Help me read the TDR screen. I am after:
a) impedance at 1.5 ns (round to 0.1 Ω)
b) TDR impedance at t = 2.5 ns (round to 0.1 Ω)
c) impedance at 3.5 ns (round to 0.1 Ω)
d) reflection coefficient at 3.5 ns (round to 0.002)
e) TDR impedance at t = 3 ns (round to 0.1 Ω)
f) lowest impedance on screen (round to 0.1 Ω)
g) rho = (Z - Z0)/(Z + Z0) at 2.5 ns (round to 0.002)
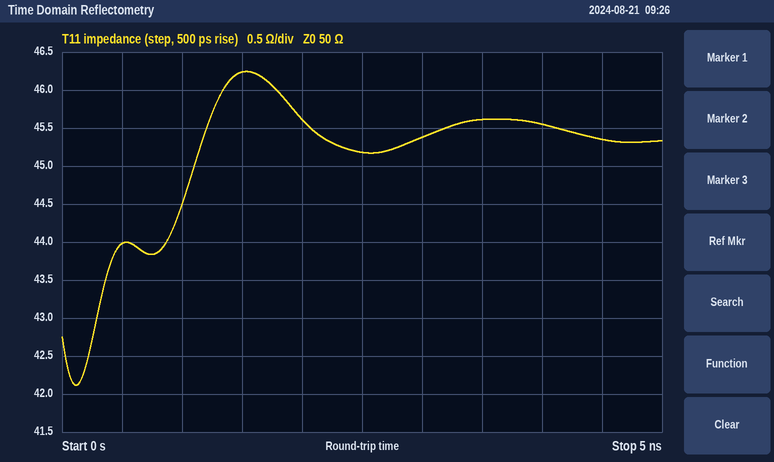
46.2 Ω
45.2 Ω
45.6 Ω
-0.046
45.4 Ω
42.1 Ω
-0.050
